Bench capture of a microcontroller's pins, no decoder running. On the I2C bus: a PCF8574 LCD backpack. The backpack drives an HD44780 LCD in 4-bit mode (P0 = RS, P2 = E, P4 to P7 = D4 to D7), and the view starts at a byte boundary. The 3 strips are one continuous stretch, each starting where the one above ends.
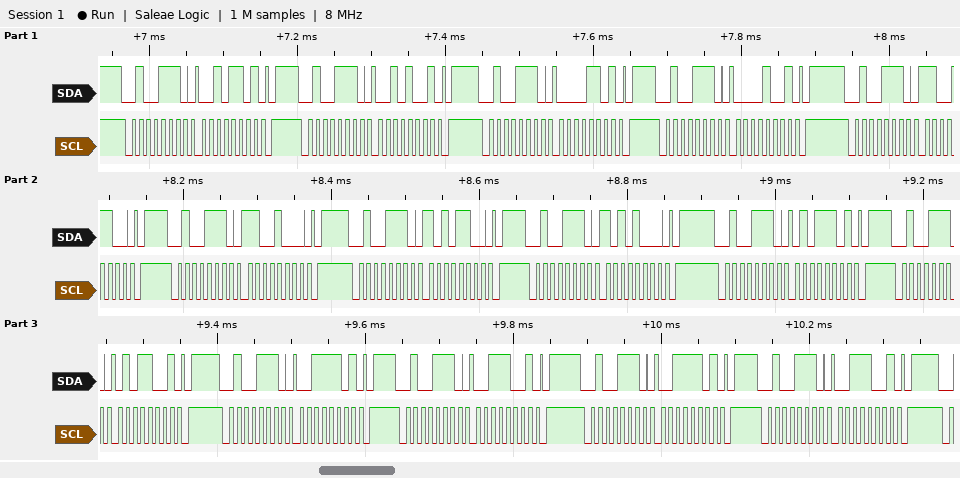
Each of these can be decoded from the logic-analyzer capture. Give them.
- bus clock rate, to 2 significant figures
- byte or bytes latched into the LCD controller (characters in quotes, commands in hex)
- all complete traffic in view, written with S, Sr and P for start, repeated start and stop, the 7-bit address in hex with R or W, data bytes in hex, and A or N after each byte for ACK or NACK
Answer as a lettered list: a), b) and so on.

a) 100 kHz
b) ' ' 0xCA 'S'
c) S 27W A 2D A P S 27W A 29 A P S 27W A 0D A P S 27W A 09 A P S 27W A CC A P S 27W A C8 A P S 27W A AC A P S 27W A A8 A P S 27W A 5D A P S 27W A 59 A P S 27W A 3D A P S 27W A 39 A P S 27W A 3D A P S 27W A 39 A P
